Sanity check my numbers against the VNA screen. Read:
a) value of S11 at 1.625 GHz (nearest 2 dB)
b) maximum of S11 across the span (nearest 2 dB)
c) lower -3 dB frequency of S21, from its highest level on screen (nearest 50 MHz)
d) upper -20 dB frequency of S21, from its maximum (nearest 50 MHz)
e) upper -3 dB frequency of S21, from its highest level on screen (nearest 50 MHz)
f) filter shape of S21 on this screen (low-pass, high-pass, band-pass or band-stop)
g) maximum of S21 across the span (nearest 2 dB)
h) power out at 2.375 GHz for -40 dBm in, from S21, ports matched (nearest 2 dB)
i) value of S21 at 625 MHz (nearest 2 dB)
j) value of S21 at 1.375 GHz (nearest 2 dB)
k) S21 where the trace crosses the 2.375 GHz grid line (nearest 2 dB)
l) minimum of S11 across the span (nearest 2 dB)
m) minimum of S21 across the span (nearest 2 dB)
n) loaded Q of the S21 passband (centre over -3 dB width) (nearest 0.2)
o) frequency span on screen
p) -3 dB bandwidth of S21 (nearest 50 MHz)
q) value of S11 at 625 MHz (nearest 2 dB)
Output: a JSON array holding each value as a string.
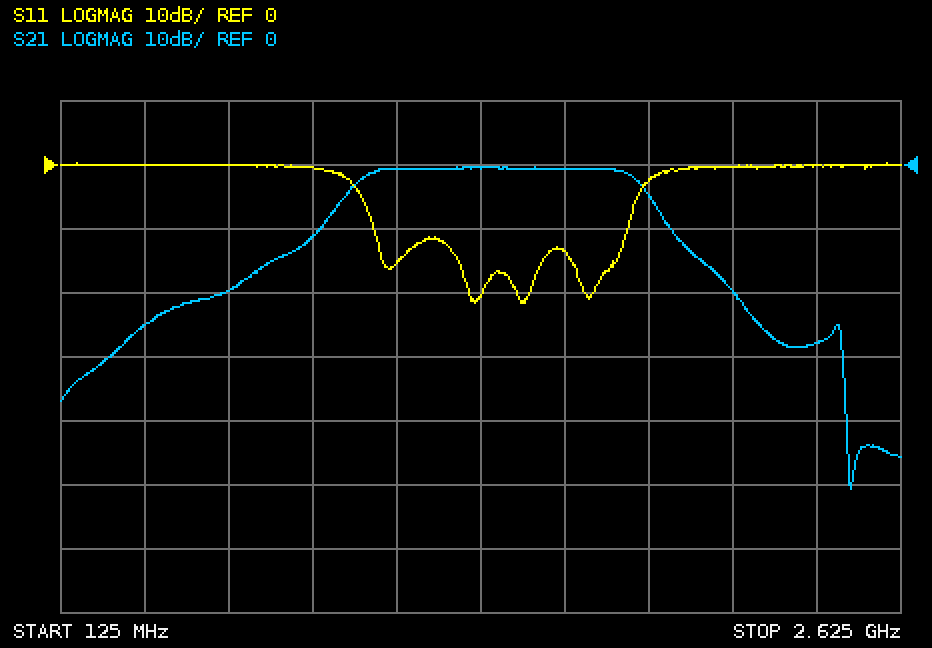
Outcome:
["-14 dB", "0 dB", "1.00 GHz", "2.15 GHz", "1.85 GHz", "band-pass", "0 dB", "-68 dBm", "-20 dB", "0 dB", "-28 dB", "-22 dB", "-50 dB", "1.6", "2.5 GHz", "850 MHz", "0 dB"]
